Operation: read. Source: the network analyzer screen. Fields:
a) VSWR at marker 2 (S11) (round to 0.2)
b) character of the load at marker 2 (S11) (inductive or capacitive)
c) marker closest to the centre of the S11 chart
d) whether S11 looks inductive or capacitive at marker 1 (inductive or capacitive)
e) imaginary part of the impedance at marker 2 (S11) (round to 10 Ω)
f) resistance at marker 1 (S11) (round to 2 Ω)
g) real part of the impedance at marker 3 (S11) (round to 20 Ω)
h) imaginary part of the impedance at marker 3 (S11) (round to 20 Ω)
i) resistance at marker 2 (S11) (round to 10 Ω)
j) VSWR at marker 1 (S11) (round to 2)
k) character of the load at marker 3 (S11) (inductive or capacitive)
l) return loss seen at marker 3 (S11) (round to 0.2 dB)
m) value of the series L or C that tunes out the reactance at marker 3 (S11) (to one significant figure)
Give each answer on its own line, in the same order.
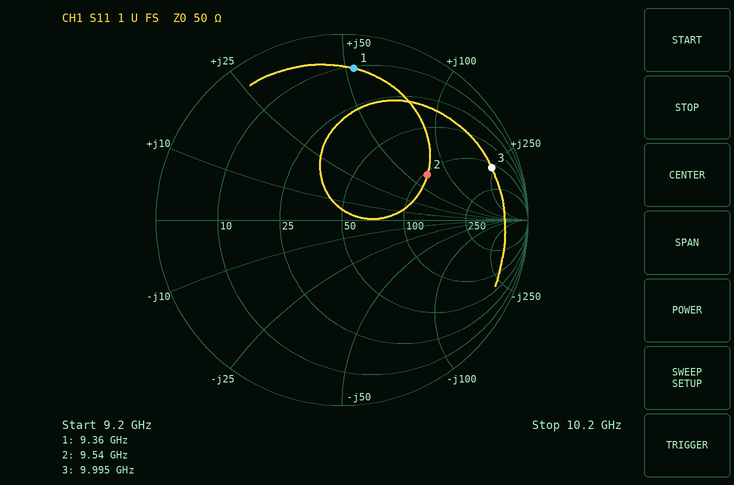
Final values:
3.2
inductive
marker 2
inductive
+70 Ω
10 Ω
120 Ω
+240 Ω
100 Ω
10
inductive
1.4 dB
70 fF
